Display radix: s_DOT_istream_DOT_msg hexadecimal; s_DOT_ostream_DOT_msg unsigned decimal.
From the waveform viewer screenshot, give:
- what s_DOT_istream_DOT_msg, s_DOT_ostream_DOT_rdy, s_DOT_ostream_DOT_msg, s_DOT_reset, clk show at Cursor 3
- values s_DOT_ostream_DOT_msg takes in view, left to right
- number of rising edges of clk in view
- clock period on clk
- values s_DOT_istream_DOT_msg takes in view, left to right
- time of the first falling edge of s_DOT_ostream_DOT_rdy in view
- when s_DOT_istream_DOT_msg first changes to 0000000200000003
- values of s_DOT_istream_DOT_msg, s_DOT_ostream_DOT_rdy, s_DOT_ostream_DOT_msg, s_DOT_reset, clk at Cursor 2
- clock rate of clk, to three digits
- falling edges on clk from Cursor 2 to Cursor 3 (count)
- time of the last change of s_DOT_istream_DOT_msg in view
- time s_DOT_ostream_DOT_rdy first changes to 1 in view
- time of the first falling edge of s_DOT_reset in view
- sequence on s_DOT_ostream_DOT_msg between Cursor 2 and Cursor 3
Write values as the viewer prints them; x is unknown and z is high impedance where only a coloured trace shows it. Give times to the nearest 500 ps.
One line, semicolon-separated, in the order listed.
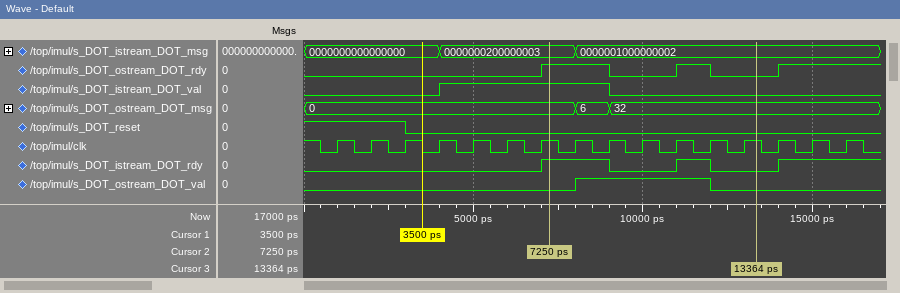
s_DOT_istream_DOT_msg=0000001000000002, s_DOT_ostream_DOT_rdy=0, s_DOT_ostream_DOT_msg=32, s_DOT_reset=0, clk=1; 0, 6, 32; 16; 1000 ps; 0000000000000000, 0000000200000003, 0000001000000002; 9000 ps; 4000 ps; s_DOT_istream_DOT_msg=0000000200000003, s_DOT_ostream_DOT_rdy=1, s_DOT_ostream_DOT_msg=0, s_DOT_reset=0, clk=1; 1.00 GHz; 6; 8000 ps; 7000 ps; 3000 ps; 0, 6, 32
